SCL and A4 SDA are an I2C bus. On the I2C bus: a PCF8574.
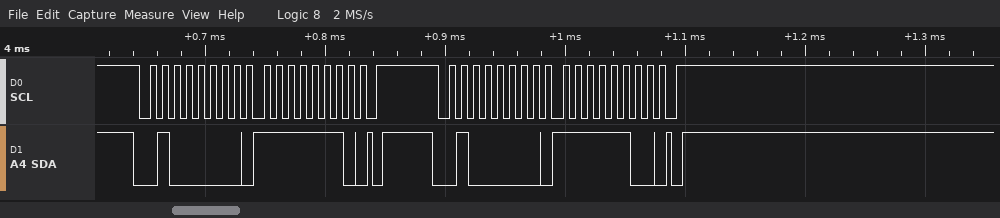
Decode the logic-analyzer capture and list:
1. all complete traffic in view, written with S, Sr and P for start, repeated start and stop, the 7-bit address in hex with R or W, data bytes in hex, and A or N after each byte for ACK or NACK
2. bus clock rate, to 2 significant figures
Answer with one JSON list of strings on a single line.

["S 20W A FE A P S 20W A FC A P", "100 kHz"]
